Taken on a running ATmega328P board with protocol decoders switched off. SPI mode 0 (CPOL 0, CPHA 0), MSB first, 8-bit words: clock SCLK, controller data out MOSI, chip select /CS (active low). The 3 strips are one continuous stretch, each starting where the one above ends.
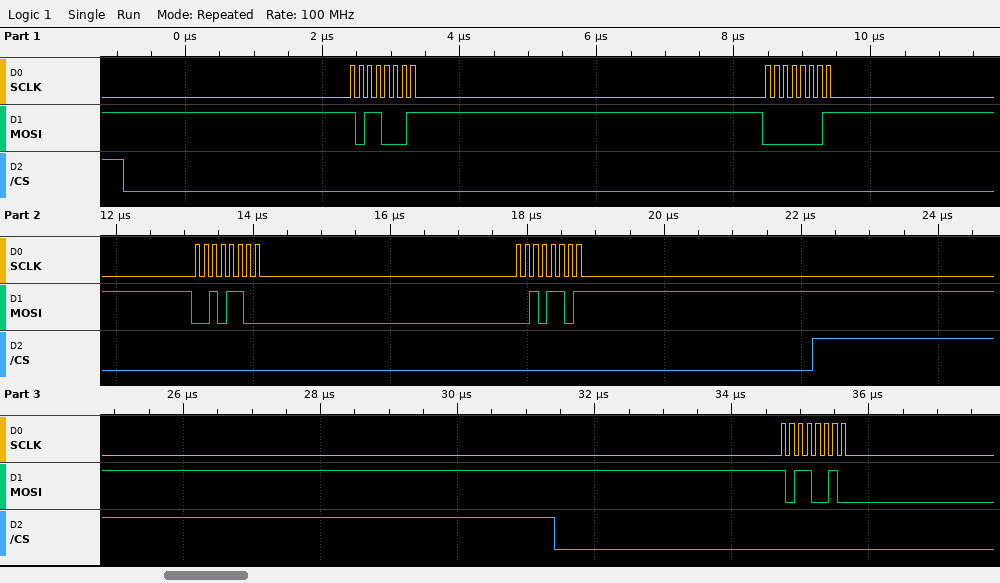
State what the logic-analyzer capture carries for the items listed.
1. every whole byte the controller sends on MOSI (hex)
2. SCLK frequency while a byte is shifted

B1 01 2C 2D B2
8 MHz
